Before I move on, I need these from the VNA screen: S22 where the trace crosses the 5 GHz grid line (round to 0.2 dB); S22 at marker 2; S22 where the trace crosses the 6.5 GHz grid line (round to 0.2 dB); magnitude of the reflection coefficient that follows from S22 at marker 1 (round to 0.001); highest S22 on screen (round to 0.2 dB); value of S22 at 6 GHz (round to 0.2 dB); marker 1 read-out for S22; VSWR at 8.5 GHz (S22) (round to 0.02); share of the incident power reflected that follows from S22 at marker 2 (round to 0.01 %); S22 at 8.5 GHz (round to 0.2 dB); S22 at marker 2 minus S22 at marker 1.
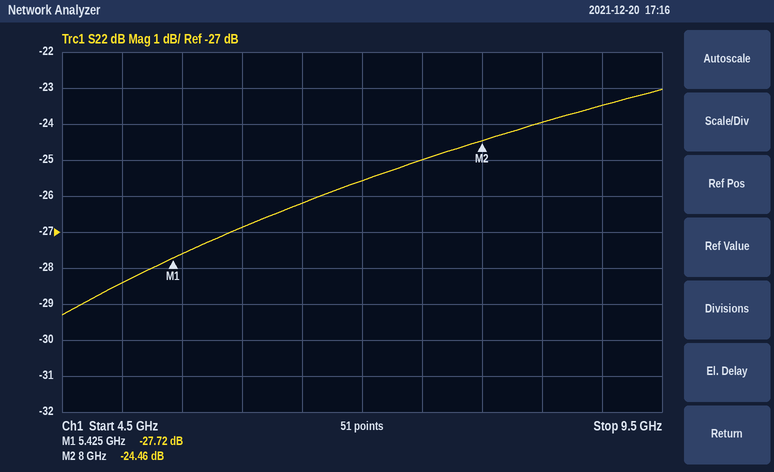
-28.4 dB
-24.46 dB
-26.2 dB
0.041
-23.0 dB
-26.8 dB
-27.72 dB
1.14
0.36 %
-24.0 dB
3.26 dB
